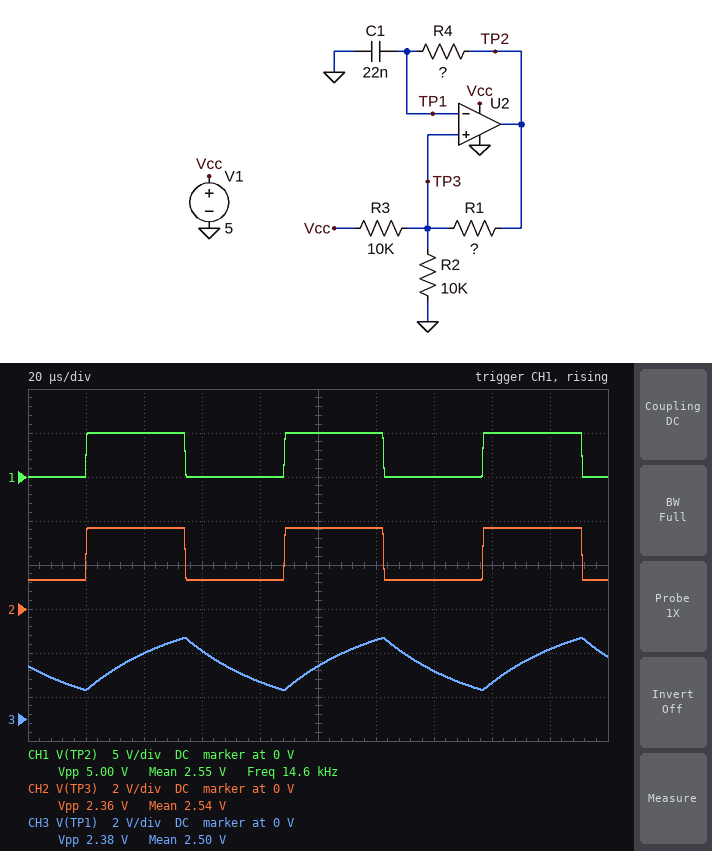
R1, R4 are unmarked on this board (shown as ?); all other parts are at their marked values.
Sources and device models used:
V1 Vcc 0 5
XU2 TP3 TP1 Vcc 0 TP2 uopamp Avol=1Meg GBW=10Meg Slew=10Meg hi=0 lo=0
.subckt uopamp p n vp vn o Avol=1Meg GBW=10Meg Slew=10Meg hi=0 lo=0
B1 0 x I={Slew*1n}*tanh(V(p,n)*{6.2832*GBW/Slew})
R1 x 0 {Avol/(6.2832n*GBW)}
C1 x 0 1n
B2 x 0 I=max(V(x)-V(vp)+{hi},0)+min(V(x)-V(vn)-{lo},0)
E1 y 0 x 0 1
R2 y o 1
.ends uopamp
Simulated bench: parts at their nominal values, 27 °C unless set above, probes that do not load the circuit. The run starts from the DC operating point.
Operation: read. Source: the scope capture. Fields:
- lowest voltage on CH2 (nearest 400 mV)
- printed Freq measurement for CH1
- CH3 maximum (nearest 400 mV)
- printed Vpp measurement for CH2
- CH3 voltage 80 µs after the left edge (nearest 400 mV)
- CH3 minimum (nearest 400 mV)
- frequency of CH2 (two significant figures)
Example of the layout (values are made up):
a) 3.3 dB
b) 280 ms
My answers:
a) 1.2 V
b) 14.6 kHz
c) 3.6 V
d) 2.36 V
e) 1.6 V
f) 1.2 V
g) 15 kHz
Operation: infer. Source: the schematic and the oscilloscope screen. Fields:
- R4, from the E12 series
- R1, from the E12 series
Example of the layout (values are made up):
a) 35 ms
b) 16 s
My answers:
a) 1.5 kΩ
b) 5.6 kΩ
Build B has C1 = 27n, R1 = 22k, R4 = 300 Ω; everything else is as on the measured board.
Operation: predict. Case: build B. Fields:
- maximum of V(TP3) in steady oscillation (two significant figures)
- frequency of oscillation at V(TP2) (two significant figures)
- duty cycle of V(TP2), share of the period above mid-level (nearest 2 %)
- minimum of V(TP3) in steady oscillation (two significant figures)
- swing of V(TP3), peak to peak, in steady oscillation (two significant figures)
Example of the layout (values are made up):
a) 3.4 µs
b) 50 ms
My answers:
a) 3.0 V
b) 140 kHz
c) 50 %
d) 2.0 V
e) 930 mV
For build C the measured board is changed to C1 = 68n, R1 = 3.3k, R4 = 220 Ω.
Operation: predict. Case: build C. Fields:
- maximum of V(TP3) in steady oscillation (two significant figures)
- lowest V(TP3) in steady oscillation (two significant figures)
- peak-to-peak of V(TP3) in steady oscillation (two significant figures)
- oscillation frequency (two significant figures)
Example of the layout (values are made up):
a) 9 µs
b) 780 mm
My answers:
a) 4.0 V
b) 990 mV
c) 3.0 V
d) 24 kHz
